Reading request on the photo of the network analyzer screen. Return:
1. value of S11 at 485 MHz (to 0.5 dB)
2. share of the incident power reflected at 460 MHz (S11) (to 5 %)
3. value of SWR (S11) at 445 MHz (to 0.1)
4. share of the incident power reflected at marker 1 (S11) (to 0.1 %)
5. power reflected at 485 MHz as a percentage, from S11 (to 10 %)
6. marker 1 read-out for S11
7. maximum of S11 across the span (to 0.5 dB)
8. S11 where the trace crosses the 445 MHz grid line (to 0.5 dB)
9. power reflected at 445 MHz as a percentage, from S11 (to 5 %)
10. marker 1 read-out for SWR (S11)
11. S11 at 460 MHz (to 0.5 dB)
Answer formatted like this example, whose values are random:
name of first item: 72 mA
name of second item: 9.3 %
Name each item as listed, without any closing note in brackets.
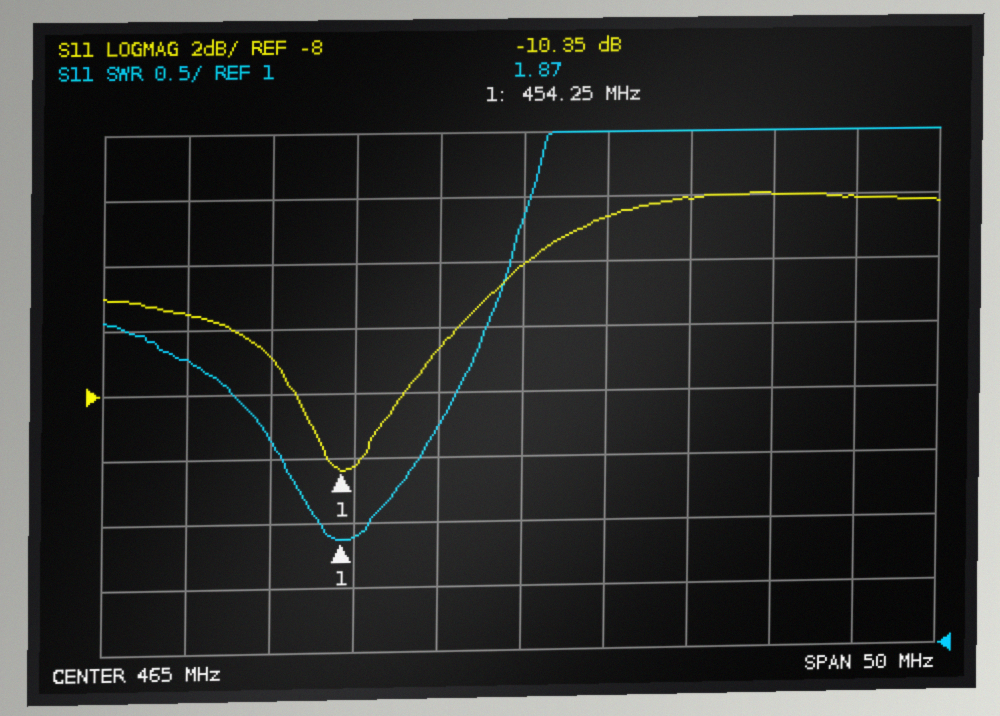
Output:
value of S11 at 485 MHz: -2.0 dB
share of the incident power reflected at 460 MHz (S11): 20 %
value of SWR (S11) at 445 MHz: 3.3
share of the incident power reflected at marker 1 (S11): 9.2 %
power reflected at 485 MHz as a percentage, from S11: 60 %
marker 1 read-out for S11: -10.35 dB
maximum of S11 across the span: -2.0 dB
S11 where the trace crosses the 445 MHz grid line: -5.5 dB
power reflected at 445 MHz as a percentage, from S11: 30 %
marker 1 read-out for SWR: 1.87
S11 at 460 MHz: -6.5 dB
